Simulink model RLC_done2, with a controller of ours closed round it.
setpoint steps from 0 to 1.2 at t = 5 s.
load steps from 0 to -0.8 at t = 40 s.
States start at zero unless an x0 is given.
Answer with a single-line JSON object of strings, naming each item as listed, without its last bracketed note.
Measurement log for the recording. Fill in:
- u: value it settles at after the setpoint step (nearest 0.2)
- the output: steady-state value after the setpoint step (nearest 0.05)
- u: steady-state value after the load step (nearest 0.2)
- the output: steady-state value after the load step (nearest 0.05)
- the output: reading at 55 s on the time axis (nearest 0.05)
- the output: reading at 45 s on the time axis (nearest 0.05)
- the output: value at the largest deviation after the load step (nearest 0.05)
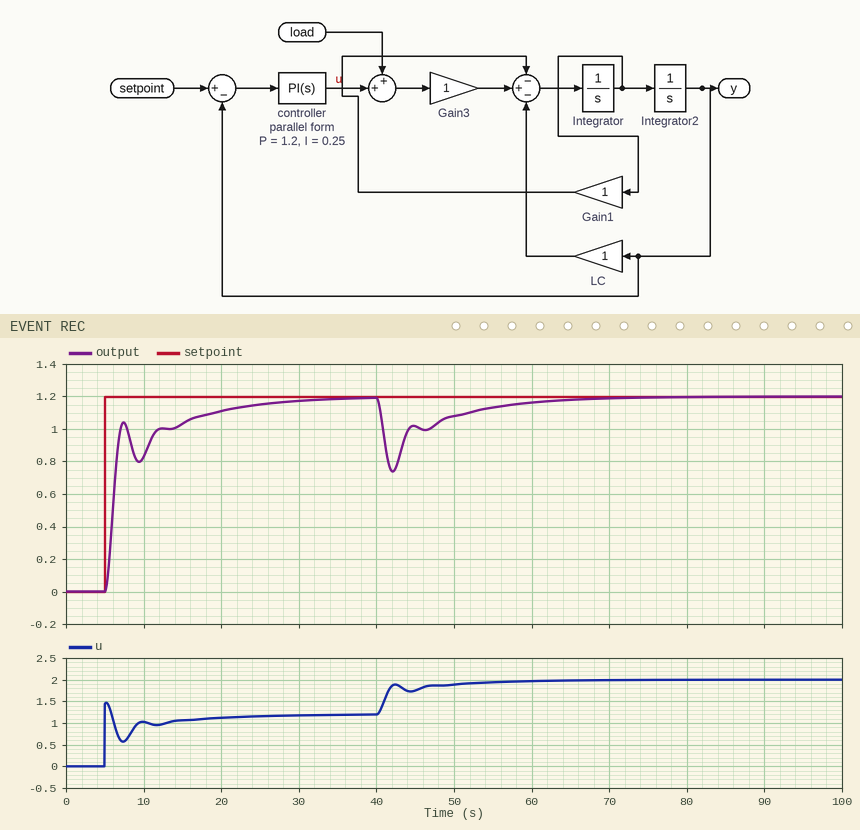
{"u: value it settles at after the setpoint step": "1.2", "the output: steady-state value after the setpoint step": "1.20", "u: steady-state value after the load step": "2.0", "the output: steady-state value after the load step": "1.20", "the output: reading at 55 s on the time axis": "1.15", "the output: reading at 45 s on the time axis": "1.00", "the output: value at the largest deviation after the load step": "0.75"}
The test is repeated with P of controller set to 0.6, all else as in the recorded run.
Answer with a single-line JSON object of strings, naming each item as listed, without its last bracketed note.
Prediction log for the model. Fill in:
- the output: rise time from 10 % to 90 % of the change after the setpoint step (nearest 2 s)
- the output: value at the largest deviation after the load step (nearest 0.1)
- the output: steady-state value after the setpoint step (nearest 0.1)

{"the output: rise time from 10 % to 90 % of the change after the setpoint step": "10 s", "the output: value at the largest deviation after the load step": "0.6", "the output: steady-state value after the setpoint step": "1.2"}
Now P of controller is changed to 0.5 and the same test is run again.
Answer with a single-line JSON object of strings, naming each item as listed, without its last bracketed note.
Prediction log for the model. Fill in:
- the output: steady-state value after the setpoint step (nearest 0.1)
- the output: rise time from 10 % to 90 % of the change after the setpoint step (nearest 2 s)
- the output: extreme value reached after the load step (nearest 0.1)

{"the output: steady-state value after the setpoint step": "1.2", "the output: rise time from 10 % to 90 % of the change after the setpoint step": "10 s", "the output: extreme value reached after the load step": "0.6"}
